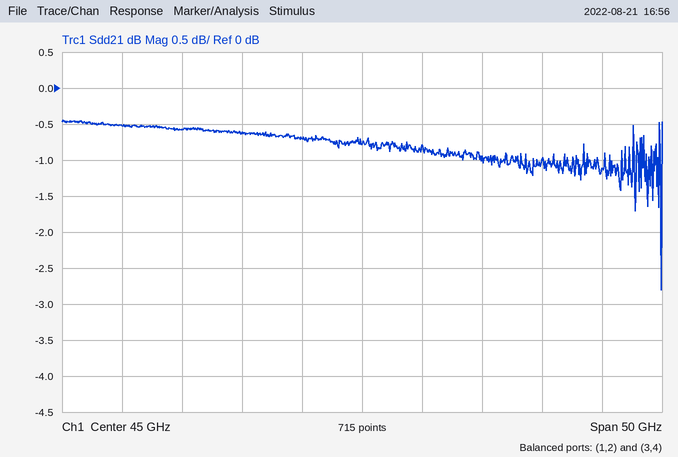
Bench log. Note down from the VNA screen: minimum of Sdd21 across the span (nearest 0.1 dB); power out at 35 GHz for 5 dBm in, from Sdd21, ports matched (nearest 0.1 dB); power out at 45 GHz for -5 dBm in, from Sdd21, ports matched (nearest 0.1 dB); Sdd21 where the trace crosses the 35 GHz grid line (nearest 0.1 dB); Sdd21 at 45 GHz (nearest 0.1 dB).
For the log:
-2.8 dB
4.4 dBm
-5.8 dBm
-0.6 dB
-0.8 dB
